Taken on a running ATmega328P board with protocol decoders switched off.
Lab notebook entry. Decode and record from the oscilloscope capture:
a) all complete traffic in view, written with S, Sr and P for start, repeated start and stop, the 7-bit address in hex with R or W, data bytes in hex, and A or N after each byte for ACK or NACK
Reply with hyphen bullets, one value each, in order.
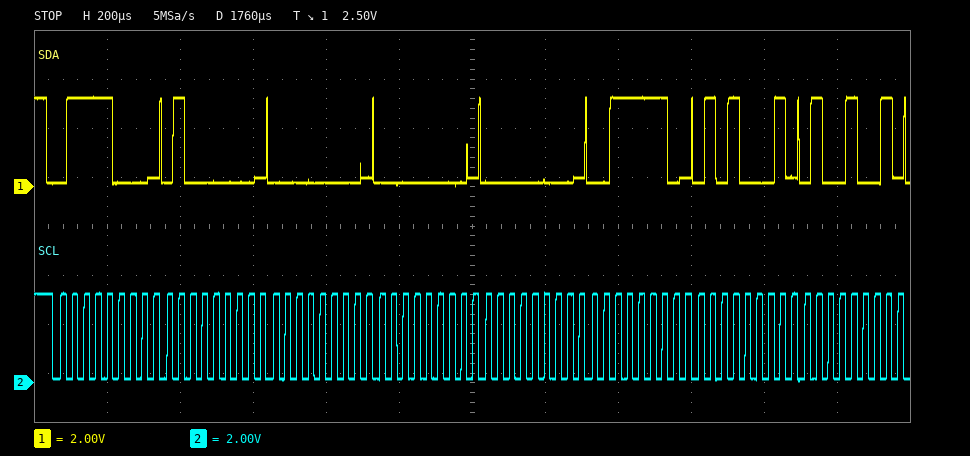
- S 3CW A 40 A 00 A 00 A 00 A 3E A 51 A 49 A
